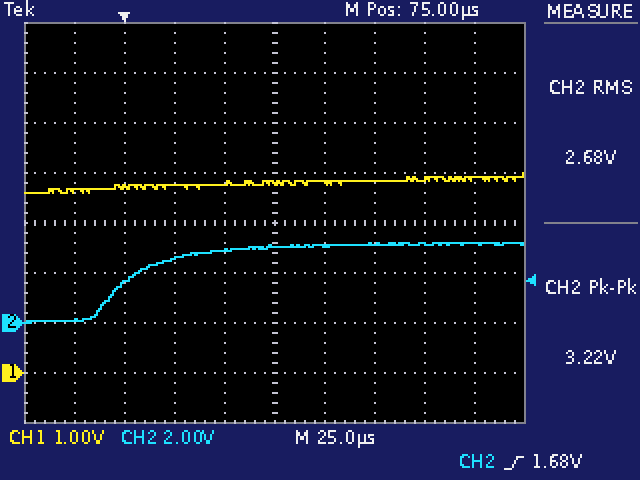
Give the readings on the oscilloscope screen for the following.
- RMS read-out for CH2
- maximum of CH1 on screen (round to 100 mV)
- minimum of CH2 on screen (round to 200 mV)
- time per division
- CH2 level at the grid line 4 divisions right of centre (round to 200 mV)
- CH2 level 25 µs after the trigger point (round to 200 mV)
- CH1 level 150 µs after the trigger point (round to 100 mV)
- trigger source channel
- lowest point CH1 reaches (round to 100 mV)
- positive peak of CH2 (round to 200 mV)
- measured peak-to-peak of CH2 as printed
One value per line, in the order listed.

2.68 V
4.0 V
0.0 V
25 µs
3.2 V
2.6 V
3.9 V
CH2
3.6 V
3.2 V
3.22 V
